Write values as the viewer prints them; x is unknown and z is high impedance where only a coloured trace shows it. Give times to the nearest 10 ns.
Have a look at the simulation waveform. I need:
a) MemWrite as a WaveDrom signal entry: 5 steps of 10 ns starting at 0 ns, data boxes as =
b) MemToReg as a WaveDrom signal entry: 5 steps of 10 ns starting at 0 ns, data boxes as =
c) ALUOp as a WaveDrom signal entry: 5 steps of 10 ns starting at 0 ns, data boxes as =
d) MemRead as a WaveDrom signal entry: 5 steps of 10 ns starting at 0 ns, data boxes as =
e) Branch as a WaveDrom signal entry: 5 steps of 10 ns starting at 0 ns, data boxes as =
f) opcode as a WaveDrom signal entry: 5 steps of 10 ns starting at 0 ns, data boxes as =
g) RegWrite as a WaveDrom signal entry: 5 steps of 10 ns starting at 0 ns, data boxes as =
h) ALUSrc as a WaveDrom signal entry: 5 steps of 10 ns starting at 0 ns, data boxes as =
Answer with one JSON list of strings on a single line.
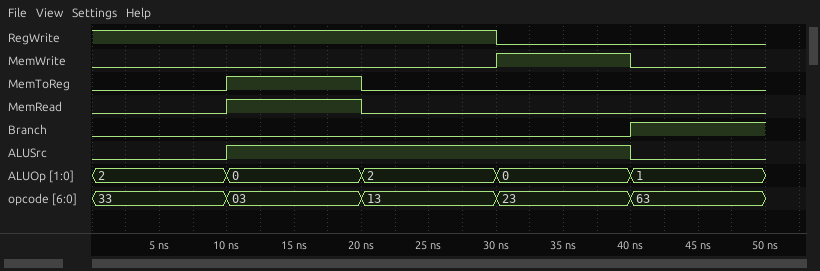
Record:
["{name: 'MemWrite', wave: '0..10'}", "{name: 'MemToReg', wave: '010..'}", "{name: 'ALUOp', wave: '=====', data: '2 0 2 0 1'}", "{name: 'MemRead', wave: '010..'}", "{name: 'Branch', wave: '0...1'}", "{name: 'opcode', wave: '=====', data: '33 03 13 23 63'}", "{name: 'RegWrite', wave: '1..0.'}", "{name: 'ALUSrc', wave: '01..0'}"]
